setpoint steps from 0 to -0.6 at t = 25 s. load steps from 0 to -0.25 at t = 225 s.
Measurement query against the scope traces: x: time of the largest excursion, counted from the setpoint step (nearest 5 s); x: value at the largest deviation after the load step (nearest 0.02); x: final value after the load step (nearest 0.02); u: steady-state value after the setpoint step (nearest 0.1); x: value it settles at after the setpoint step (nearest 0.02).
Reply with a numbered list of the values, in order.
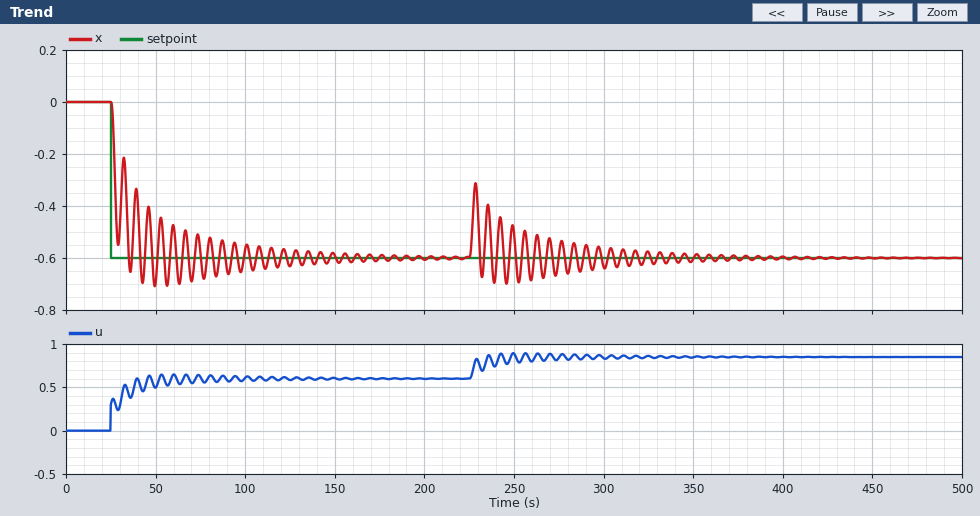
1. 25 s
2. -0.32
3. -0.60
4. 0.6
5. -0.60
